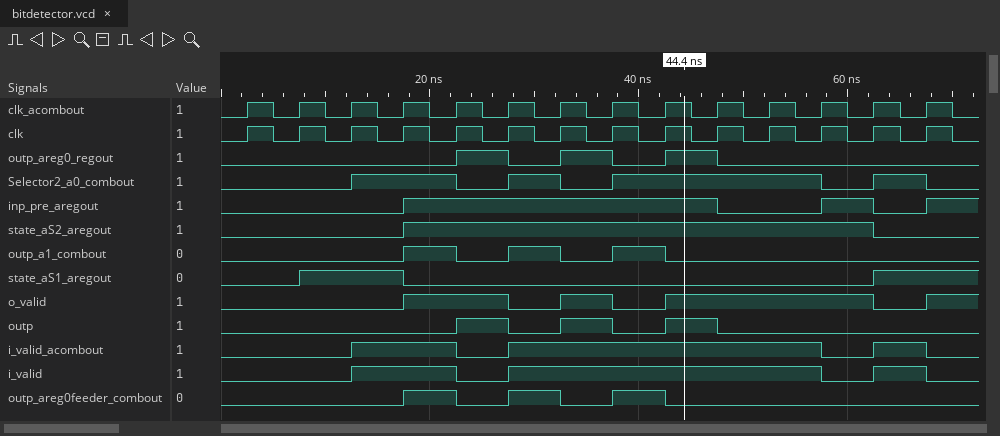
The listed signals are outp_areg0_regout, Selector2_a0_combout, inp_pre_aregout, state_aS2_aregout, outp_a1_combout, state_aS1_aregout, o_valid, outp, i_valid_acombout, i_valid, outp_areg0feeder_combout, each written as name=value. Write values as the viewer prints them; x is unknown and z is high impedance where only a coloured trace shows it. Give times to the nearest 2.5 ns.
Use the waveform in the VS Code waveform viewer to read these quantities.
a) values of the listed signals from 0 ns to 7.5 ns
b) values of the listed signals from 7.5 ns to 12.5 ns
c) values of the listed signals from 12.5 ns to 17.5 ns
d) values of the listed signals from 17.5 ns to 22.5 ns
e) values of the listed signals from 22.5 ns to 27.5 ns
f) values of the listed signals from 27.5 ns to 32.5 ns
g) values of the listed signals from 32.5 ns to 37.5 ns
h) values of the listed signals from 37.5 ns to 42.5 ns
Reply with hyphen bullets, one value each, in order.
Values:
- outp_areg0_regout=0, Selector2_a0_combout=0, inp_pre_aregout=0, state_aS2_aregout=0, outp_a1_combout=0, state_aS1_aregout=0, o_valid=0, outp=0, i_valid_acombout=0, i_valid=0, outp_areg0feeder_combout=0
- outp_areg0_regout=0, Selector2_a0_combout=0, inp_pre_aregout=0, state_aS2_aregout=0, outp_a1_combout=0, state_aS1_aregout=1, o_valid=0, outp=0, i_valid_acombout=0, i_valid=0, outp_areg0feeder_combout=0
- outp_areg0_regout=0, Selector2_a0_combout=1, inp_pre_aregout=0, state_aS2_aregout=0, outp_a1_combout=0, state_aS1_aregout=1, o_valid=0, outp=0, i_valid_acombout=1, i_valid=1, outp_areg0feeder_combout=0
- outp_areg0_regout=0, Selector2_a0_combout=1, inp_pre_aregout=1, state_aS2_aregout=1, outp_a1_combout=1, state_aS1_aregout=0, o_valid=1, outp=0, i_valid_acombout=1, i_valid=1, outp_areg0feeder_combout=1
- outp_areg0_regout=1, Selector2_a0_combout=0, inp_pre_aregout=1, state_aS2_aregout=1, outp_a1_combout=0, state_aS1_aregout=0, o_valid=1, outp=1, i_valid_acombout=0, i_valid=0, outp_areg0feeder_combout=0
- outp_areg0_regout=0, Selector2_a0_combout=1, inp_pre_aregout=1, state_aS2_aregout=1, outp_a1_combout=1, state_aS1_aregout=0, o_valid=0, outp=0, i_valid_acombout=1, i_valid=1, outp_areg0feeder_combout=1
- outp_areg0_regout=1, Selector2_a0_combout=0, inp_pre_aregout=1, state_aS2_aregout=1, outp_a1_combout=0, state_aS1_aregout=0, o_valid=1, outp=1, i_valid_acombout=1, i_valid=1, outp_areg0feeder_combout=0
- outp_areg0_regout=0, Selector2_a0_combout=1, inp_pre_aregout=1, state_aS2_aregout=1, outp_a1_combout=1, state_aS1_aregout=0, o_valid=0, outp=0, i_valid_acombout=1, i_valid=1, outp_areg0feeder_combout=1
